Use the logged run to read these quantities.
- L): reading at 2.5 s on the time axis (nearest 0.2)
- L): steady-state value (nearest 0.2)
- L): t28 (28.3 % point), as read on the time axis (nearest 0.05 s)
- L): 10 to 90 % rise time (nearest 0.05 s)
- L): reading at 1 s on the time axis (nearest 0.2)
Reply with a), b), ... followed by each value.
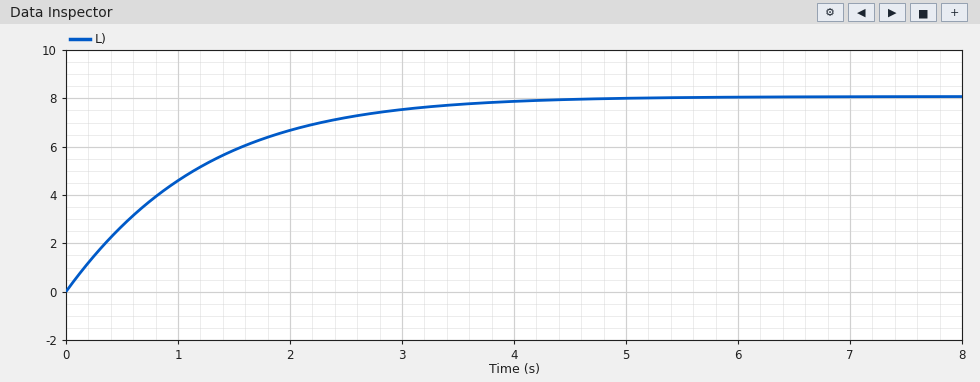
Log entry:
a) 7.2
b) 8.0
c) 0.40 s
d) 2.45 s
e) 4.6
